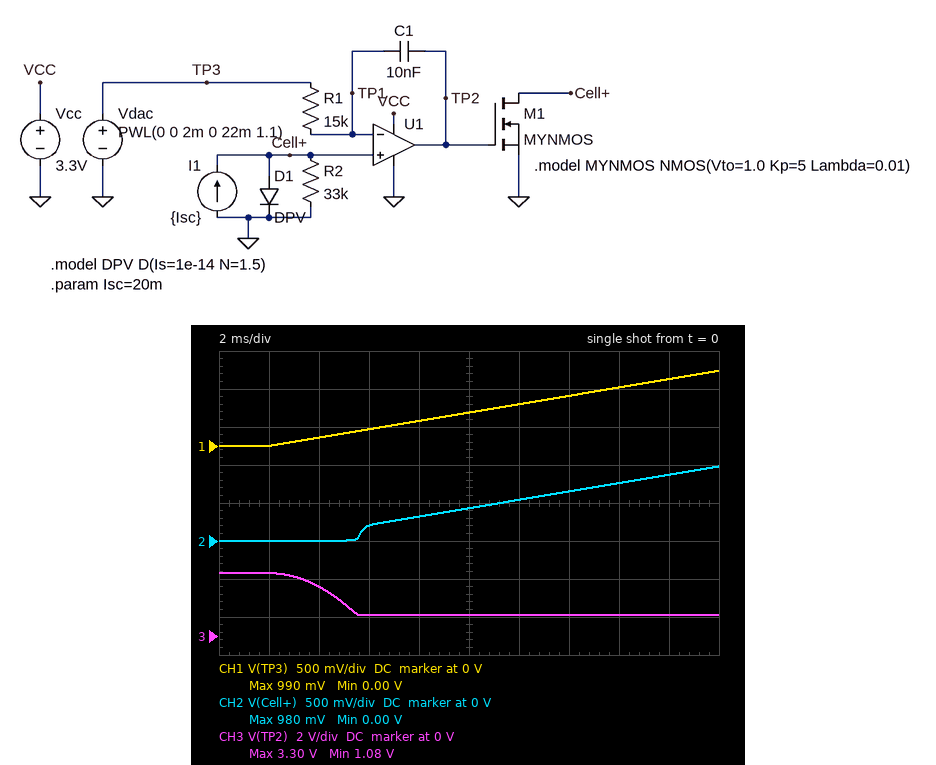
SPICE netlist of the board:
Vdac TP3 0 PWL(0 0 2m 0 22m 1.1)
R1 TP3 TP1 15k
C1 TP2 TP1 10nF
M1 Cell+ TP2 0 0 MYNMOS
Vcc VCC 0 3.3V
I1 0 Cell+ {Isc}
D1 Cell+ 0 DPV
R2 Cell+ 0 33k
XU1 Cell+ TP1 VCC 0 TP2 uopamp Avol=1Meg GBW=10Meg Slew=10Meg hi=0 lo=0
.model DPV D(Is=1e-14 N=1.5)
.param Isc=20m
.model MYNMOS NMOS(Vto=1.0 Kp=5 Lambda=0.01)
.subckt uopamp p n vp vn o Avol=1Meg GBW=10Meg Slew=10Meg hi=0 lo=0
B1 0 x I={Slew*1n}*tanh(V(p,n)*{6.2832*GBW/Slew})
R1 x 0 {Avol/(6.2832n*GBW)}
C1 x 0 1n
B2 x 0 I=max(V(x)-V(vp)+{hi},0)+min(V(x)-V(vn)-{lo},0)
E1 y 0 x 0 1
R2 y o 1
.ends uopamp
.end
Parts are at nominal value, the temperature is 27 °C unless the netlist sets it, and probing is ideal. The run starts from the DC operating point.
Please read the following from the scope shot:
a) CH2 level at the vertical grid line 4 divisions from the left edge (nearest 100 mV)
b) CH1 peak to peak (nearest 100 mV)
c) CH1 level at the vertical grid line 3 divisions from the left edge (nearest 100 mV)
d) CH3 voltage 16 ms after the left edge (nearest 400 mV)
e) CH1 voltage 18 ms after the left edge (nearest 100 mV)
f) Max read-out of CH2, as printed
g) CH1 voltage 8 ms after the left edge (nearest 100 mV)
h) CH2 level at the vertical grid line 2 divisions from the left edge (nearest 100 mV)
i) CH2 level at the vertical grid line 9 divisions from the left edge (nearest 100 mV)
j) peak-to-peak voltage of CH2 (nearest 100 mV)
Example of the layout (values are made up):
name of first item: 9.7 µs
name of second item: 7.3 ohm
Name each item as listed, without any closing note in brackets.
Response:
CH2 level at the vertical grid line 4 divisions from the left edge: 300 mV
CH1 peak to peak: 1.0 V
CH1 level at the vertical grid line 3 divisions from the left edge: 200 mV
CH3 voltage 16 ms after the left edge: 1.2 V
CH1 voltage 18 ms after the left edge: 900 mV
Max read-out of CH2, as printed: 980 mV
CH1 voltage 8 ms after the left edge: 300 mV
CH2 level at the vertical grid line 2 divisions from the left edge: 0 V
CH2 level at the vertical grid line 9 divisions from the left edge: 900 mV
peak-to-peak voltage of CH2: 1.0 V
